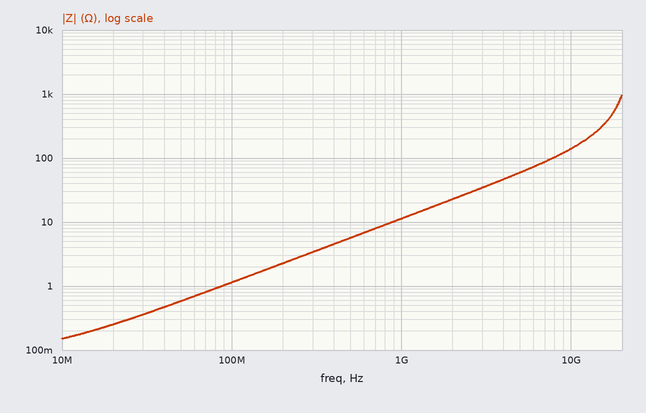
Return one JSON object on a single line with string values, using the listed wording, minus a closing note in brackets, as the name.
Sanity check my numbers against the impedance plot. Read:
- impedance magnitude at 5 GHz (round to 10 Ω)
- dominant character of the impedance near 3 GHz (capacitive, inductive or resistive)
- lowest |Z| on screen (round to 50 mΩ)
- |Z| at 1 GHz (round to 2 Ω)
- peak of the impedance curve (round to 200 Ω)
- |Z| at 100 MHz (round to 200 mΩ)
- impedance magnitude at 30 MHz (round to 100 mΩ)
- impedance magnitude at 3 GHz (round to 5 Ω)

{"impedance magnitude at 5 GHz": "60 Ω", "dominant character of the impedance near 3 GHz": "inductive", "lowest |Z| on screen": "150 mΩ", "|Z| at 1 GHz": "12 Ω", "peak of the impedance curve": "1.0 kΩ", "|Z| at 100 MHz": "1.2 Ω", "impedance magnitude at 30 MHz": "400 mΩ", "impedance magnitude at 3 GHz": "35 Ω"}
